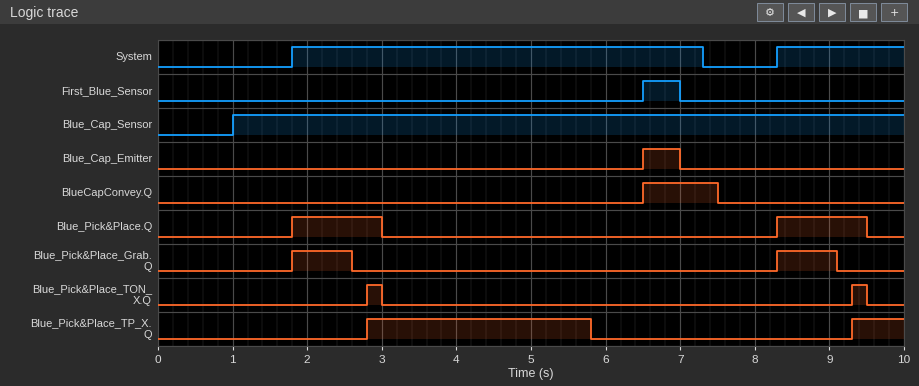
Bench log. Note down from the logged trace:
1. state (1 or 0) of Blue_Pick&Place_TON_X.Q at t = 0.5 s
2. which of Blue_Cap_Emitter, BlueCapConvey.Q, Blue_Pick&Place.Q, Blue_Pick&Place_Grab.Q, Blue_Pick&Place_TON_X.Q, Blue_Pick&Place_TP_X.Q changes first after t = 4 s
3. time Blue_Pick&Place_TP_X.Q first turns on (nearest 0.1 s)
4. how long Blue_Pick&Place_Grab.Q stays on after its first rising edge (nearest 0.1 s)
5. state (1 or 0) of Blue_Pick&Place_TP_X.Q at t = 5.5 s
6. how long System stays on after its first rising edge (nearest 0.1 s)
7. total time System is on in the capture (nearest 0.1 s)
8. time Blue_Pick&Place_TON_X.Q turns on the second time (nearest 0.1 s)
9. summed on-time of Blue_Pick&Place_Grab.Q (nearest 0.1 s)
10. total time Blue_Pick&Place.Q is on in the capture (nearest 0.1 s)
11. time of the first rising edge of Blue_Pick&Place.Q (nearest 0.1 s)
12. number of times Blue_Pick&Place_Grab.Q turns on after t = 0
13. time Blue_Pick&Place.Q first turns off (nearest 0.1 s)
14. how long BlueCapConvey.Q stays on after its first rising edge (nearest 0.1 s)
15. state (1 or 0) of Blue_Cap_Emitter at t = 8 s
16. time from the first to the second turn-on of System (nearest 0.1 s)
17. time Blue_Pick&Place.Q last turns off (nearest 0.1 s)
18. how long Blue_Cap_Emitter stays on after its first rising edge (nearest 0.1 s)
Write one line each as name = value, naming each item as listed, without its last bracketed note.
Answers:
state (1 or 0) of Blue_Pick&Place_TON_X.Q at t = 0.5 s = 0
which of Blue_Cap_Emitter, BlueCapConvey.Q, Blue_Pick&Place.Q, Blue_Pick&Place_Grab.Q, Blue_Pick&Place_TON_X.Q, Blue_Pick&Place_TP_X.Q changes first after t = 4 s = Blue_Pick&Place_TP_X.Q
time Blue_Pick&Place_TP_X.Q first turns on = 2.8 s
how long Blue_Pick&Place_Grab.Q stays on after its first rising edge = 0.8 s
state (1 or 0) of Blue_Pick&Place_TP_X.Q at t = 5.5 s = 1
how long System stays on after its first rising edge = 5.5 s
total time System is on in the capture = 7.2 s
time Blue_Pick&Place_TON_X.Q turns on the second time = 9.3 s
summed on-time of Blue_Pick&Place_Grab.Q = 1.6 s
total time Blue_Pick&Place.Q is on in the capture = 2.4 s
time of the first rising edge of Blue_Pick&Place.Q = 1.8 s
number of times Blue_Pick&Place_Grab.Q turns on after t = 0 = 2
time Blue_Pick&Place.Q first turns off = 3.0 s
how long BlueCapConvey.Q stays on after its first rising edge = 1.0 s
state (1 or 0) of Blue_Cap_Emitter at t = 8 s = 0
time from the first to the second turn-on of System = 6.5 s
time Blue_Pick&Place.Q last turns off = 9.5 s
how long Blue_Cap_Emitter stays on after its first rising edge = 0.5 s
